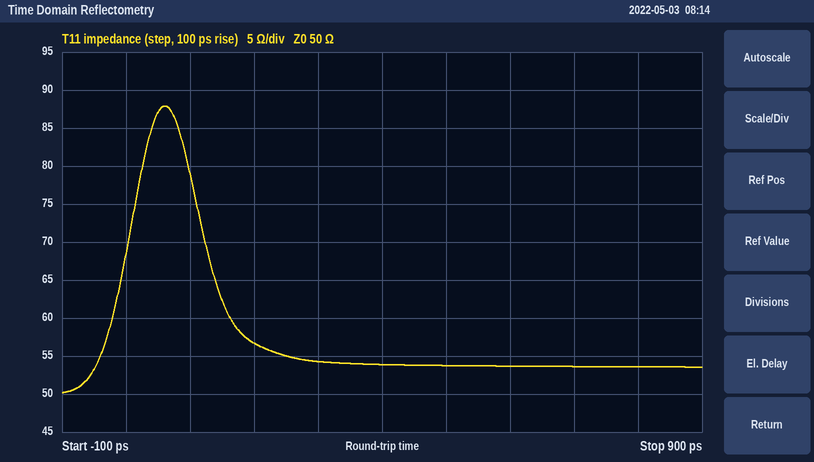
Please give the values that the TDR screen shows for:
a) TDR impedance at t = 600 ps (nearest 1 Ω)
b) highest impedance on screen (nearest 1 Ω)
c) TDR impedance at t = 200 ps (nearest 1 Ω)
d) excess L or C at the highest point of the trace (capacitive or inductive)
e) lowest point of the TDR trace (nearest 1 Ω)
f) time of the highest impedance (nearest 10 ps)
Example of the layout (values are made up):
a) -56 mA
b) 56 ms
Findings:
a) 54 Ω
b) 88 Ω
c) 57 Ω
d) inductive
e) 50 Ω
f) 60 ps
